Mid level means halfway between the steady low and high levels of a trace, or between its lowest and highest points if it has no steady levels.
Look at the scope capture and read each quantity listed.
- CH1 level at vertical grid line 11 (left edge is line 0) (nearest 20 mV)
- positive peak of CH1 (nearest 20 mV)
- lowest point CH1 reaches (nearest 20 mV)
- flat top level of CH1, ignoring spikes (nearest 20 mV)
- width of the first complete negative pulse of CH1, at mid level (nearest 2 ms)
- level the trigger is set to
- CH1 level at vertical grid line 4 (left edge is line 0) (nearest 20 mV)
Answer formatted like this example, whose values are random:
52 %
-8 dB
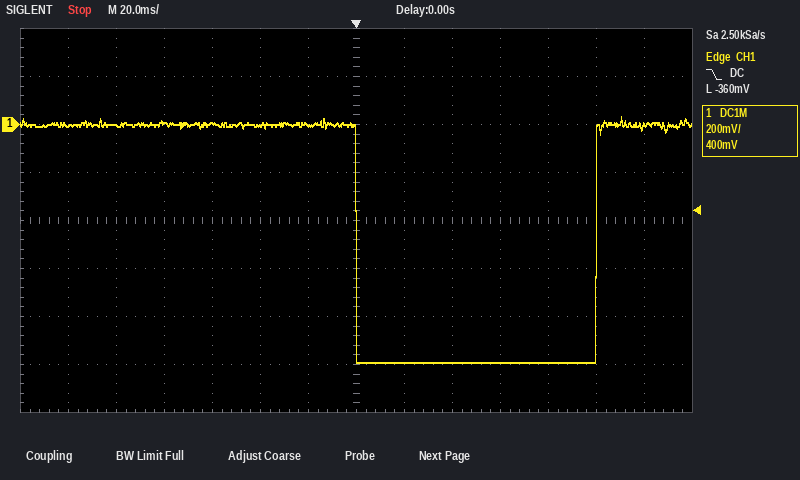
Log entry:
-1.00 V
40 mV
-1.00 V
0 mV
100 ms
-360 mV
0 mV
